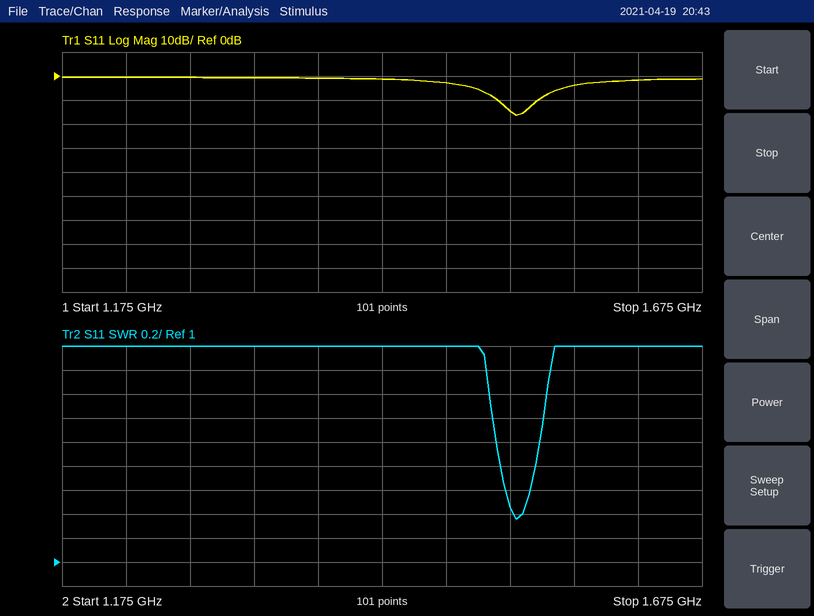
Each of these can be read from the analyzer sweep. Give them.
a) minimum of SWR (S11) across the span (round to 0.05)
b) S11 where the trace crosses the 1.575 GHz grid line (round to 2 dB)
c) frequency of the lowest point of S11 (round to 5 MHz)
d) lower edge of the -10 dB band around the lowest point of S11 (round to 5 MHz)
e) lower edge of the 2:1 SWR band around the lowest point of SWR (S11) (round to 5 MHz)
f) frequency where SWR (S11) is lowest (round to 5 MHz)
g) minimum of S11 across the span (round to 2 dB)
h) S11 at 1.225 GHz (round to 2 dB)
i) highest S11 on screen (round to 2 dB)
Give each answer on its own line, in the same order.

1.35
-4 dB
1.530 GHz
1.515 GHz
1.515 GHz
1.530 GHz
-16 dB
0 dB
0 dB
